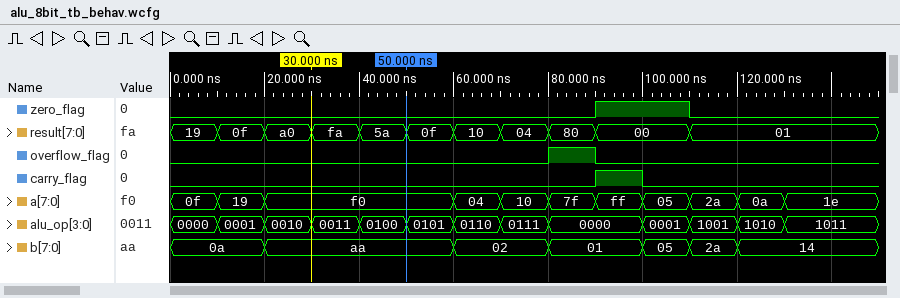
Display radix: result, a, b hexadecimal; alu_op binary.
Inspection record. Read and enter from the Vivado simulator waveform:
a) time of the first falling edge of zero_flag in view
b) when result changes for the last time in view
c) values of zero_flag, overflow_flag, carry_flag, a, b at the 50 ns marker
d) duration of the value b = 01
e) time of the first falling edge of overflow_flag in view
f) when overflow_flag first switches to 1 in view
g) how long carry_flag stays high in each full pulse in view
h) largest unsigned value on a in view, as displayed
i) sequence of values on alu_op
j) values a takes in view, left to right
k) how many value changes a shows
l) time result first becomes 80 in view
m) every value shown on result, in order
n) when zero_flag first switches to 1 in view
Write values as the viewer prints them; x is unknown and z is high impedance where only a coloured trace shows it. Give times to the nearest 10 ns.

110 ns
110 ns
zero_flag=0, overflow_flag=0, carry_flag=0, a=f0, b=aa
20 ns
90 ns
80 ns
10 ns
ff
0000, 0001, 0010, 0011, 0100, 0101, 0110, 0111, 0000, 0001, 1001, 1010, 1011
0f, 19, f0, 04, 10, 7f, ff, 05, 2a, 0a, 1e
10
80 ns
19, 0f, a0, fa, 5a, 0f, 10, 04, 80, 00, 01
90 ns
